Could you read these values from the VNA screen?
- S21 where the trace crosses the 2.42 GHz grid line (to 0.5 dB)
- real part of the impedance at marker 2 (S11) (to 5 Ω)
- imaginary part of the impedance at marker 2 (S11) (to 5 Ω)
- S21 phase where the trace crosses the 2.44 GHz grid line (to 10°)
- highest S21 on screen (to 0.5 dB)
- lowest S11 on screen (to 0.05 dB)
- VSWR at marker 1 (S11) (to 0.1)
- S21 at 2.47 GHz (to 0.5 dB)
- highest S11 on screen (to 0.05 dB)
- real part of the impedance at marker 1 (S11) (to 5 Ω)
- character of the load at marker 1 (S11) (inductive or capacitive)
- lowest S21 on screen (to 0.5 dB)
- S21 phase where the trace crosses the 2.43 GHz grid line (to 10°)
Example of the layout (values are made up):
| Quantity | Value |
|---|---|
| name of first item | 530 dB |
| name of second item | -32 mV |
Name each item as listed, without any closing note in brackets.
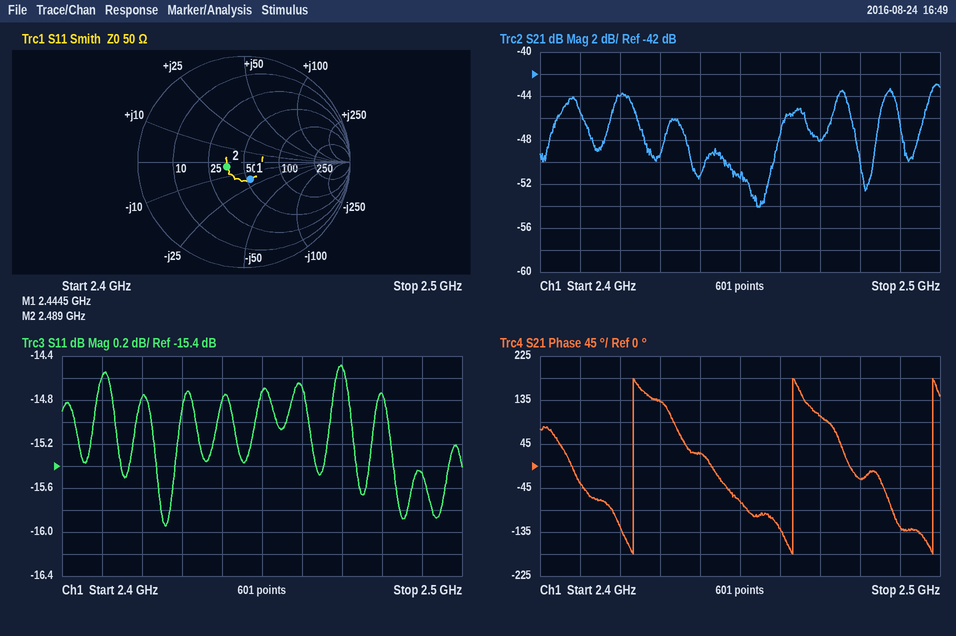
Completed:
| Quantity | Value |
|---|---|
| S21 where the trace crosses the 2.42 GHz grid line | -44.0 dB |
| real part of the impedance at marker 2 (S11) | 35 Ω |
| imaginary part of the impedance at marker 2 (S11) | -5 Ω |
| S21 phase where the trace crosses the 2.44 GHz grid line | 30° |
| highest S21 on screen | -43.0 dB |
| lowest S11 on screen | -15.95 dB |
| VSWR at marker 1 (S11) | 1.4 |
| S21 at 2.47 GHz | -48.0 dB |
| highest S11 on screen | -14.50 dB |
| real part of the impedance at marker 1 (S11) | 55 Ω |
| character of the load at marker 1 (S11) | capacitive |
| lowest S21 on screen | -54.0 dB |
| S21 phase where the trace crosses the 2.43 GHz grid line | 130° |
